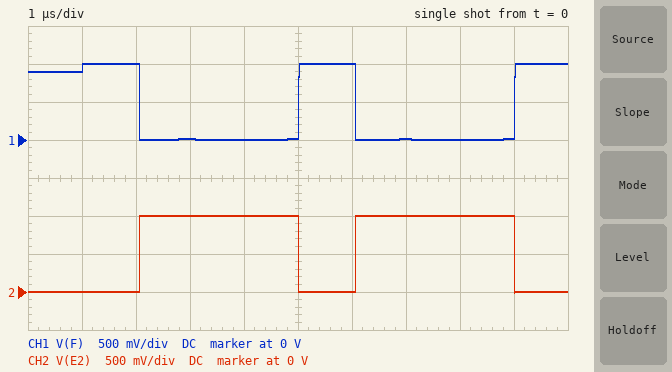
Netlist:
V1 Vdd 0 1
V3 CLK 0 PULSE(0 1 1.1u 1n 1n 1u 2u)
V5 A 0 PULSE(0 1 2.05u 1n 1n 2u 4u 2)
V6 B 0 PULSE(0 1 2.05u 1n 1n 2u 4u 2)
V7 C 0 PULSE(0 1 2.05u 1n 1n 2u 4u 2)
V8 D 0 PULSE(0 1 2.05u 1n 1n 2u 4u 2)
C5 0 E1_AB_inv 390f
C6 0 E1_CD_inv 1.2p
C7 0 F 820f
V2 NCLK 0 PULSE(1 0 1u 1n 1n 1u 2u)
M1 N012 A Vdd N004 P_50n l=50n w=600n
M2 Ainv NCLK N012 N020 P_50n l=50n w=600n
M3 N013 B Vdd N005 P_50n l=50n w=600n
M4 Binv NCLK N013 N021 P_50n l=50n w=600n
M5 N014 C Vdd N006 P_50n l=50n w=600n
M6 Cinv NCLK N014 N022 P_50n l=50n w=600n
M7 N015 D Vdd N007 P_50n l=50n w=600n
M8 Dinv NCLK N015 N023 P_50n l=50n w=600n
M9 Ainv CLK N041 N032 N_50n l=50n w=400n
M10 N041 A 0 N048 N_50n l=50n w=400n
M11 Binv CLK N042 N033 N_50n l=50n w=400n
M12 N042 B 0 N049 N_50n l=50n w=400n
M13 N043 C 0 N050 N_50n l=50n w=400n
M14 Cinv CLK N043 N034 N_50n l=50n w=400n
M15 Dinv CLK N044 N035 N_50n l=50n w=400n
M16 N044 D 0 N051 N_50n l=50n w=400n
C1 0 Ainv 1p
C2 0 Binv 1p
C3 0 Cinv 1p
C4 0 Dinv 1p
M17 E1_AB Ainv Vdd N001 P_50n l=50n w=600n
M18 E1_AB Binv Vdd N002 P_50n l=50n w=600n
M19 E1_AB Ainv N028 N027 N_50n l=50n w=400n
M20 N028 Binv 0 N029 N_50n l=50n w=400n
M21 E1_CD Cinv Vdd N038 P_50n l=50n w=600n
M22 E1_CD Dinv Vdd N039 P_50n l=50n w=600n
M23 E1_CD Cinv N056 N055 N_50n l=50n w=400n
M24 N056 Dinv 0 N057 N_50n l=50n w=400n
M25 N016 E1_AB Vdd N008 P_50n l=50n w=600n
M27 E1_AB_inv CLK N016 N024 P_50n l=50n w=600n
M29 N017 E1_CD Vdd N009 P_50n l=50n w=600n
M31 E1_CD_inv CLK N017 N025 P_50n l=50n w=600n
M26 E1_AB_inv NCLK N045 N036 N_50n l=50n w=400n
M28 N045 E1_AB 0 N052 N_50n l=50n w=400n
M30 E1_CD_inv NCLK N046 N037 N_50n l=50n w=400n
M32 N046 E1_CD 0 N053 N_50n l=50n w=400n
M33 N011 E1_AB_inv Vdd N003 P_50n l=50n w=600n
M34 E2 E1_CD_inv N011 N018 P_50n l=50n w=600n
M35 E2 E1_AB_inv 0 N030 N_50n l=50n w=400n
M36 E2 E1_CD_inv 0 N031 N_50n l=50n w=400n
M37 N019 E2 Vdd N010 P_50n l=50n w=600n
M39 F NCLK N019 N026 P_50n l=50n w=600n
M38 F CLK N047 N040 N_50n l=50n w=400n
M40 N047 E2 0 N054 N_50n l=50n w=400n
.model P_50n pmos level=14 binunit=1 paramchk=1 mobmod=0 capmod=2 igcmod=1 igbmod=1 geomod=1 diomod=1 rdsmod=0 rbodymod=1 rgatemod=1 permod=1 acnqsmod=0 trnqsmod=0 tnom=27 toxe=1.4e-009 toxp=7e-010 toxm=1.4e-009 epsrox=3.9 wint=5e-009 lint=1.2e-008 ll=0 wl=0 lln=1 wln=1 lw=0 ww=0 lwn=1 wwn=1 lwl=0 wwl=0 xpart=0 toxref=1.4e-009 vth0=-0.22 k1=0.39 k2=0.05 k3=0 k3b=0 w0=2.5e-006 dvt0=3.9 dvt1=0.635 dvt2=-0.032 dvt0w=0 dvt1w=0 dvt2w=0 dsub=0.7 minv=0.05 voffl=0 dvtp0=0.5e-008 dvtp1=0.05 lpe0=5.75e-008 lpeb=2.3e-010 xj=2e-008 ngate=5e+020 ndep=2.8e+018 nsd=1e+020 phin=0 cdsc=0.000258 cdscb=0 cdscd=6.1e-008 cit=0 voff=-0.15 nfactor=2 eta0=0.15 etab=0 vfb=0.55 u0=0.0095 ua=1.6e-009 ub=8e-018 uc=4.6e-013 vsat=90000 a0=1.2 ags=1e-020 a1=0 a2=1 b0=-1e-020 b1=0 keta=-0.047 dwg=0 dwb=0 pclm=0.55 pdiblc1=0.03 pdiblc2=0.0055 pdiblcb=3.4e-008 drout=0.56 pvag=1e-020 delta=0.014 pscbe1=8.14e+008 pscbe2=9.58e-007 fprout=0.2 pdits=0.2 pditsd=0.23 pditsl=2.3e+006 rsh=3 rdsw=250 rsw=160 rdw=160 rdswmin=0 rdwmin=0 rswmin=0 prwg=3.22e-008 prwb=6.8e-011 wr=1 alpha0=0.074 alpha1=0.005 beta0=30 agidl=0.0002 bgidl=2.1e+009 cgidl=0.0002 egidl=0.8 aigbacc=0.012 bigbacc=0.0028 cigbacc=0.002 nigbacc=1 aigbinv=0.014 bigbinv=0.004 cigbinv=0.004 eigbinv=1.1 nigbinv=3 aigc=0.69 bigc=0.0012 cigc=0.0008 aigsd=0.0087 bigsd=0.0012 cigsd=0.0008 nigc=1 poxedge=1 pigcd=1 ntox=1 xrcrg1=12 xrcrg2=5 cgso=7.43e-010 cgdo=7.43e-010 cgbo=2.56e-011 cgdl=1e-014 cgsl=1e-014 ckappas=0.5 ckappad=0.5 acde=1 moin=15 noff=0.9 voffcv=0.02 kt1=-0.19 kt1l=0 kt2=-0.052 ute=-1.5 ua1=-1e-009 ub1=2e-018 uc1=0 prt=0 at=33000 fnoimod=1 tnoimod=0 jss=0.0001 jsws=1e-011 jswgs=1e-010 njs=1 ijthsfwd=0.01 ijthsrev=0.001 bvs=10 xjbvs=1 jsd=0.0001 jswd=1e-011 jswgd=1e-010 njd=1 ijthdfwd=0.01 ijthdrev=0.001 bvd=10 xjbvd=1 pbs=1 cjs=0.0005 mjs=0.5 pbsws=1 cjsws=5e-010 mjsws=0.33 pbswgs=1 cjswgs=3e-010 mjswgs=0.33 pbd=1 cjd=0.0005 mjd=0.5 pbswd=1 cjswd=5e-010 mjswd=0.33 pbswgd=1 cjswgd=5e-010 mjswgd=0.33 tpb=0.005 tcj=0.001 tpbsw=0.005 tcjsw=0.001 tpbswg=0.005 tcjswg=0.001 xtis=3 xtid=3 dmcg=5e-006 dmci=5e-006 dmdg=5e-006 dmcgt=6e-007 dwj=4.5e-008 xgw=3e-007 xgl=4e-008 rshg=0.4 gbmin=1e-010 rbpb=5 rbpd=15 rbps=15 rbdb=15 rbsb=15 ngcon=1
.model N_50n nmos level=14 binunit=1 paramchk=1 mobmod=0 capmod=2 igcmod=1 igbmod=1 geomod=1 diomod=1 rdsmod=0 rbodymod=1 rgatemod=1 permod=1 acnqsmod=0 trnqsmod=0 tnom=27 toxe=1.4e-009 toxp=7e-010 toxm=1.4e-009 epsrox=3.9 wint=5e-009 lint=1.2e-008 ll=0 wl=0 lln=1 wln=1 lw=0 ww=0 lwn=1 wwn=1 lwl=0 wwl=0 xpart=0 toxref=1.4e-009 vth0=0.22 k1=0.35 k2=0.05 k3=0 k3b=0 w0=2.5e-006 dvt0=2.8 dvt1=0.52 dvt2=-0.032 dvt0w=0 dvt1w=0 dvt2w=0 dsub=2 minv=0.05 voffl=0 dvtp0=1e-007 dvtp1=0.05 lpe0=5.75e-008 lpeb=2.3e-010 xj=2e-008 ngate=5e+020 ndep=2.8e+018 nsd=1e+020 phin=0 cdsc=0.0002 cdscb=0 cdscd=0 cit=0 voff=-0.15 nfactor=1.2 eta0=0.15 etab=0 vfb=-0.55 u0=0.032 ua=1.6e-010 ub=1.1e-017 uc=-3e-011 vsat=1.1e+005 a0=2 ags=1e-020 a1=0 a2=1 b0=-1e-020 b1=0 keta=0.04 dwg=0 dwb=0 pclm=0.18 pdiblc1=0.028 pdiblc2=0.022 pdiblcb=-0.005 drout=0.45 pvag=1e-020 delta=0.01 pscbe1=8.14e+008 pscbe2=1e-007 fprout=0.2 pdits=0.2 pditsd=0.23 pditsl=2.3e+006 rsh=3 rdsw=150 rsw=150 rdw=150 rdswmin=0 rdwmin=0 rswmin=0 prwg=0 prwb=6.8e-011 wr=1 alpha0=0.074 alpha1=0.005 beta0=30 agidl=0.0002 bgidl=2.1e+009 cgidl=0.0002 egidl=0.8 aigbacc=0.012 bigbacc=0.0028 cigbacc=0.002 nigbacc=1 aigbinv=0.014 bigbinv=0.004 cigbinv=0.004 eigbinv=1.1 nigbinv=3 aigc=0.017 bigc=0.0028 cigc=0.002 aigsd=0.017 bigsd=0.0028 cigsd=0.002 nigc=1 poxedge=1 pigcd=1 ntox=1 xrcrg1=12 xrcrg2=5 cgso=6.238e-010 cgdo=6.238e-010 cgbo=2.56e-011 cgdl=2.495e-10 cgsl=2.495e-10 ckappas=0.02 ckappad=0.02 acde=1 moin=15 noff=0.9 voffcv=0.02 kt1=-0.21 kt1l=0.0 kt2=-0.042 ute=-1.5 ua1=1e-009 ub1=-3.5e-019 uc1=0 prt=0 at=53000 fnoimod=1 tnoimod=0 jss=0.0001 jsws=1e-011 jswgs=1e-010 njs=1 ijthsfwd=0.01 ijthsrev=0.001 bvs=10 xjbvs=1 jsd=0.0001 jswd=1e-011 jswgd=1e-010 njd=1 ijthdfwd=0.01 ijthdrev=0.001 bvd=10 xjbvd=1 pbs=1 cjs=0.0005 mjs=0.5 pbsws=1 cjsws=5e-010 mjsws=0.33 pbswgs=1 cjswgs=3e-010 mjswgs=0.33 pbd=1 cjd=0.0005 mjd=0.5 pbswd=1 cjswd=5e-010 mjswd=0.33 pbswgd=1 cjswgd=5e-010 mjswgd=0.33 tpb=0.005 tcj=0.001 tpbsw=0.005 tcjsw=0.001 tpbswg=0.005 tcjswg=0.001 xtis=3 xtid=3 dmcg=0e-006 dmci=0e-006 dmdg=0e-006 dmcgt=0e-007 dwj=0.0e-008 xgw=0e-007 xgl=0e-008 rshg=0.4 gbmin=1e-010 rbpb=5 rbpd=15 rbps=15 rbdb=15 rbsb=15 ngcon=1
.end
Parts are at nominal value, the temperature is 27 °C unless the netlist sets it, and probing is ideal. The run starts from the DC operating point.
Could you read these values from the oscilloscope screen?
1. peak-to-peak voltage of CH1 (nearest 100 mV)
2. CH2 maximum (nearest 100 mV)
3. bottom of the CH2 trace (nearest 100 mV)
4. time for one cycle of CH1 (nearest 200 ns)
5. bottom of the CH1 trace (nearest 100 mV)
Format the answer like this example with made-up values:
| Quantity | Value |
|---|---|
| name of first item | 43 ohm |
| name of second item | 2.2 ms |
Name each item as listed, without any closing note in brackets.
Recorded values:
| Quantity | Value |
|---|---|
| peak-to-peak voltage of CH1 | 1.0 V |
| CH2 maximum | 1.0 V |
| bottom of the CH2 trace | 0 V |
| time for one cycle of CH1 | 4.0 µs |
| bottom of the CH1 trace | 0 V |
